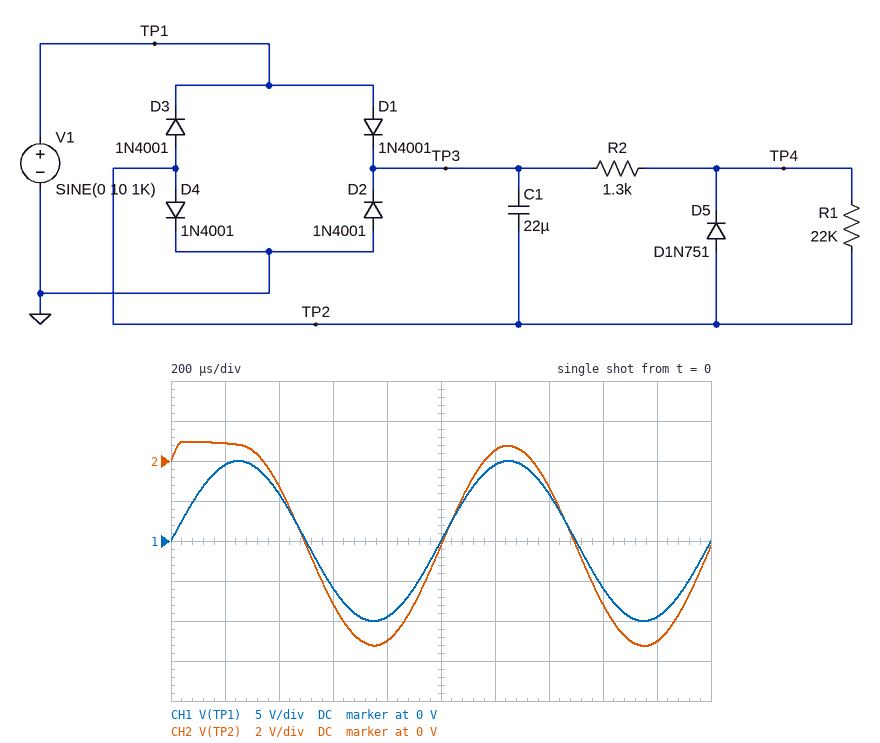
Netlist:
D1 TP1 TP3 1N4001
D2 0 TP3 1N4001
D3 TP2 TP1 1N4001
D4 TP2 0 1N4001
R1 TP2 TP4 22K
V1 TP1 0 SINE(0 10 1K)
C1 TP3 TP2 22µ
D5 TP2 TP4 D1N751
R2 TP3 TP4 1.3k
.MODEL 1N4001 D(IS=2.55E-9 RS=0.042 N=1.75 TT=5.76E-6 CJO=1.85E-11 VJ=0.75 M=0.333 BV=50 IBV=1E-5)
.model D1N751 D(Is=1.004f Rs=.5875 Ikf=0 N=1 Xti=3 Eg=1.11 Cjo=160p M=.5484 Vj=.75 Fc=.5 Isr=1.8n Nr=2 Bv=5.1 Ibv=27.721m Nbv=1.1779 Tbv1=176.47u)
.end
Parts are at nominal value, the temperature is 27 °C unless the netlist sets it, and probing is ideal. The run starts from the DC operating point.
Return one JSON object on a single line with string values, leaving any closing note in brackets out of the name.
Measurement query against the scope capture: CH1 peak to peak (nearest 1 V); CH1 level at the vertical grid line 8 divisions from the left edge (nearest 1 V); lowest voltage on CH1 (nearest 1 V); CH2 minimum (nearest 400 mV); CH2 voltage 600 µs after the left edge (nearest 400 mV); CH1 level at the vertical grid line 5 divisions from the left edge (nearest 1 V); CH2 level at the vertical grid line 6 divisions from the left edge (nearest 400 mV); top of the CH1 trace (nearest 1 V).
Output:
{"CH1 peak to peak": "20 V", "CH1 level at the vertical grid line 8 divisions from the left edge": "-6 V", "lowest voltage on CH1": "-10 V", "CH2 minimum": "-9.2 V", "CH2 voltage 600 µs after the left edge": "-7.2 V", "CH1 level at the vertical grid line 5 divisions from the left edge": "0 V", "CH2 level at the vertical grid line 6 divisions from the left edge": "400 mV", "top of the CH1 trace": "10 V"}
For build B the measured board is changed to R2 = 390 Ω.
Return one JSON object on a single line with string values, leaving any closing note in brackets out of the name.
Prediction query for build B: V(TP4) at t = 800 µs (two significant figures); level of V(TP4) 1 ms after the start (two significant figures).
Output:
{"V(TP4) at t = 800 µs": "-3.9 V", "level of V(TP4) 1 ms after the start": "890 mV"}
